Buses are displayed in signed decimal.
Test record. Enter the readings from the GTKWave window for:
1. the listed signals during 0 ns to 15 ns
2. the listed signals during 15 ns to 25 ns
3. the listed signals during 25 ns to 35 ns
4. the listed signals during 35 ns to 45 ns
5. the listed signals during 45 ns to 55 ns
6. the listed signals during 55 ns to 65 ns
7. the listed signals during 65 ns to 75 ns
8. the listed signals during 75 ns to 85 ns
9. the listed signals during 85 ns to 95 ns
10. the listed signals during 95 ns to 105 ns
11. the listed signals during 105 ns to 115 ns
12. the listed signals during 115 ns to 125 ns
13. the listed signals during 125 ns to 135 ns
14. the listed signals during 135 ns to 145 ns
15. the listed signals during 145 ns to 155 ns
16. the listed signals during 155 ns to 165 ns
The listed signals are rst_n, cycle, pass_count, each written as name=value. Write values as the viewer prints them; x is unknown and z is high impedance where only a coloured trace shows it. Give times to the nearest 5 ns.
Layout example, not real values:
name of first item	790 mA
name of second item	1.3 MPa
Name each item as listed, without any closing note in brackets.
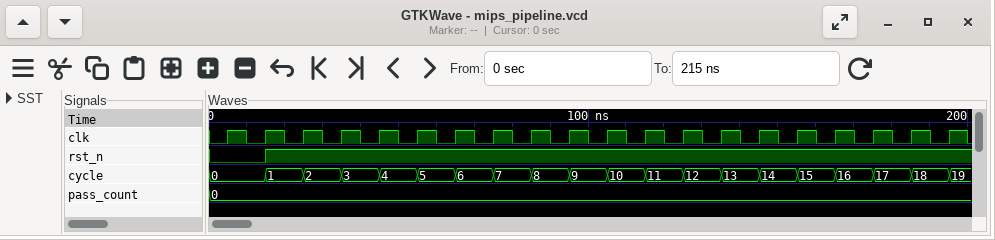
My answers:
the listed signals during 0 ns to 15 ns	rst_n=0, cycle=0, pass_count=0
the listed signals during 15 ns to 25 ns	rst_n=1, cycle=1, pass_count=0
the listed signals during 25 ns to 35 ns	rst_n=1, cycle=2, pass_count=0
the listed signals during 35 ns to 45 ns	rst_n=1, cycle=3, pass_count=0
the listed signals during 45 ns to 55 ns	rst_n=1, cycle=4, pass_count=0
the listed signals during 55 ns to 65 ns	rst_n=1, cycle=5, pass_count=0
the listed signals during 65 ns to 75 ns	rst_n=1, cycle=6, pass_count=0
the listed signals during 75 ns to 85 ns	rst_n=1, cycle=7, pass_count=0
the listed signals during 85 ns to 95 ns	rst_n=1, cycle=8, pass_count=0
the listed signals during 95 ns to 105 ns	rst_n=1, cycle=9, pass_count=0
the listed signals during 105 ns to 115 ns	rst_n=1, cycle=10, pass_count=0
the listed signals during 115 ns to 125 ns	rst_n=1, cycle=11, pass_count=0
the listed signals during 125 ns to 135 ns	rst_n=1, cycle=12, pass_count=0
the listed signals during 135 ns to 145 ns	rst_n=1, cycle=13, pass_count=0
the listed signals during 145 ns to 155 ns	rst_n=1, cycle=14, pass_count=0
the listed signals during 155 ns to 165 ns	rst_n=1, cycle=15, pass_count=0
